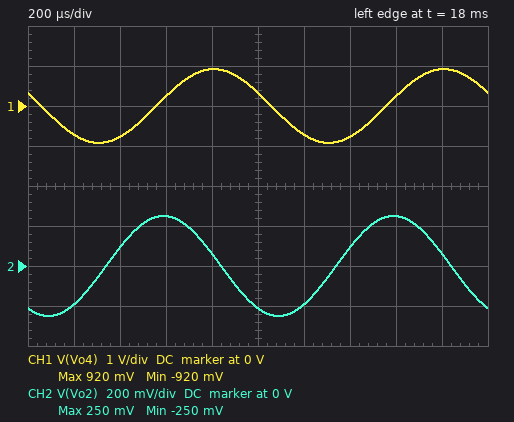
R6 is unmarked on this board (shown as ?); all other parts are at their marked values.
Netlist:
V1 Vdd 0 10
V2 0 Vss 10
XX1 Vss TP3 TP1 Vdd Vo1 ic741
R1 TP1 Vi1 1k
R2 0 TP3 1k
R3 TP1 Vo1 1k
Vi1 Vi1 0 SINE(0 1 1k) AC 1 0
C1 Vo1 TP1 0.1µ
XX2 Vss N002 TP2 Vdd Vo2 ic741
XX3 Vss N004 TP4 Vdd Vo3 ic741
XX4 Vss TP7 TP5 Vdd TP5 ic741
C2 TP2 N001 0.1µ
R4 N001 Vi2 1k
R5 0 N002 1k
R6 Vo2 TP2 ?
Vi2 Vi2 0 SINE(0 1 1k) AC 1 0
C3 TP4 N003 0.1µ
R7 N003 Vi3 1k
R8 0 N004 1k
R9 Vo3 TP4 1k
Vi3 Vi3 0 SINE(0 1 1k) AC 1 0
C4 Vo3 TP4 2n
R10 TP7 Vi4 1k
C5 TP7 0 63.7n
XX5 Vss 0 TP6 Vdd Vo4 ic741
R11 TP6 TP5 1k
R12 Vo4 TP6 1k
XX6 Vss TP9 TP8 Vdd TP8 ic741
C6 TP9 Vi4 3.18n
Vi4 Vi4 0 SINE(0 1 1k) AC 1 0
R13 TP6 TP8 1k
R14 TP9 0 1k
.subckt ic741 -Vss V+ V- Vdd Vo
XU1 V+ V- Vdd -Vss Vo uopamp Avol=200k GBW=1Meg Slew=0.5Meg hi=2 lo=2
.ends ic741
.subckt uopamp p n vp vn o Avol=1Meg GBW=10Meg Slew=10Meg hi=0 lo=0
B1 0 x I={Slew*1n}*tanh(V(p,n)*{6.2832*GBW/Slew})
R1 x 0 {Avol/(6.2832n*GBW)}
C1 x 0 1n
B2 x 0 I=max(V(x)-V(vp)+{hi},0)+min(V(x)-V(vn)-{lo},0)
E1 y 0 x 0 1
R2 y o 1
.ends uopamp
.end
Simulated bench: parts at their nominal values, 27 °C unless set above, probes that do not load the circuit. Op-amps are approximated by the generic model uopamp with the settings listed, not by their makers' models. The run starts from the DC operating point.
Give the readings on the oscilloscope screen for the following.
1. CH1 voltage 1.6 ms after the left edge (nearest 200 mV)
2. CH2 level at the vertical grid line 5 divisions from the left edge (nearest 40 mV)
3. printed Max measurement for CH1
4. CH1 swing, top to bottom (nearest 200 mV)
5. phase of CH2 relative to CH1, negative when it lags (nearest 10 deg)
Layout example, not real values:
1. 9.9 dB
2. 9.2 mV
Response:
1. 200 mV
2. -200 mV
3. 920 mV
4. 1.8 V
5. 80 deg
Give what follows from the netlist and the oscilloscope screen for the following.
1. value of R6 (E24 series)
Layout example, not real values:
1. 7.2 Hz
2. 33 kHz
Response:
1. 470 Ω
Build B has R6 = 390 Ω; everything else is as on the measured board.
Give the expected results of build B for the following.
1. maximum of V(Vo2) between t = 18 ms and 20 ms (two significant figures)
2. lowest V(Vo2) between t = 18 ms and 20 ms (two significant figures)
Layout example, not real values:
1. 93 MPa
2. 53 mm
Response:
1. 210 mV
2. -210 mV
